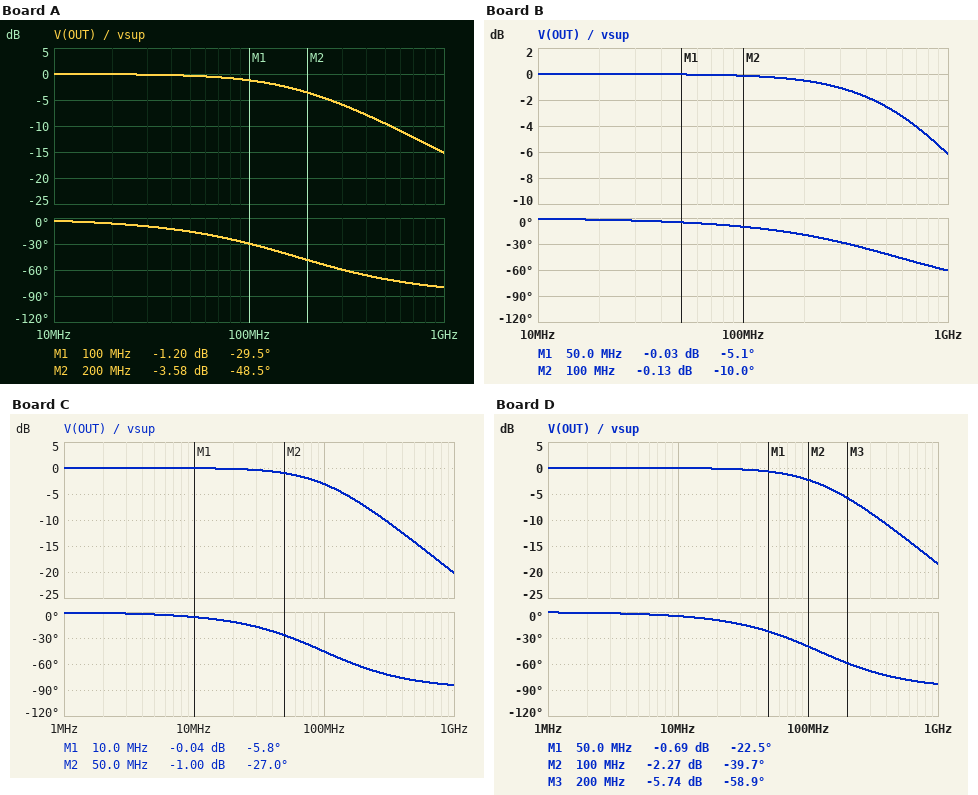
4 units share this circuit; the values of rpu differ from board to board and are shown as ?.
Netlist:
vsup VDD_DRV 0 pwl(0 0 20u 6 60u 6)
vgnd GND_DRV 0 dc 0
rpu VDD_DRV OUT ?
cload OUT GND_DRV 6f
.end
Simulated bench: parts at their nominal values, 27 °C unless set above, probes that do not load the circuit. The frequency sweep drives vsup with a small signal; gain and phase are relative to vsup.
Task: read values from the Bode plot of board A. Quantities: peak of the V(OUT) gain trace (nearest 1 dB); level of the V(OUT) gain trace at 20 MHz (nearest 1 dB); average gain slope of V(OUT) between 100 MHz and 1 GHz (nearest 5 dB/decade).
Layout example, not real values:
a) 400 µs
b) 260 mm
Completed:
a) 0 dB
b) 0 dB
c) -15 dB/decade
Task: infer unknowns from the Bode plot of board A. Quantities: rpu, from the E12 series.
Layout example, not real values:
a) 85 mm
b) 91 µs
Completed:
a) 150 kΩ
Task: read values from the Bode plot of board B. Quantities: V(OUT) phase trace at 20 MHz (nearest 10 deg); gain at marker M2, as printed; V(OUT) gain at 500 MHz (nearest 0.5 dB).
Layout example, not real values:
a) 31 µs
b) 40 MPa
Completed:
a) 0 deg
b) -0.13 dB
c) -2.5 dB
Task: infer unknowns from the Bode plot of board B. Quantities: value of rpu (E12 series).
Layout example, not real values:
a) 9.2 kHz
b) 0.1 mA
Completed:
a) 47 kΩ
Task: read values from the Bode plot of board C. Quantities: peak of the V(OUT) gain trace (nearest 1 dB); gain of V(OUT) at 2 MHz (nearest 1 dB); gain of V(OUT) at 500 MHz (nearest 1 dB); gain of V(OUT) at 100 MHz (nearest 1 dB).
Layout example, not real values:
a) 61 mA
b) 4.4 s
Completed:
a) 0 dB
b) 0 dB
c) -14 dB
d) -3 dB
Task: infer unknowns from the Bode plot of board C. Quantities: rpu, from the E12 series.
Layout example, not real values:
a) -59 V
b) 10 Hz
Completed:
a) 270 kΩ
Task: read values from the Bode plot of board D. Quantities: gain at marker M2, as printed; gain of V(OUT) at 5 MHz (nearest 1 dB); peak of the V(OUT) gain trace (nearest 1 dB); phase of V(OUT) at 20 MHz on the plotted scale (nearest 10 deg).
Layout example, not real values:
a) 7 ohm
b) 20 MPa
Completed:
a) -2.27 dB
b) 0 dB
c) 0 dB
d) -10 deg
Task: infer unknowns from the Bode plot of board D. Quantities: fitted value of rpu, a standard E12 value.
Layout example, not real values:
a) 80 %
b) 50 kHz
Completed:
a) 220 kΩ
